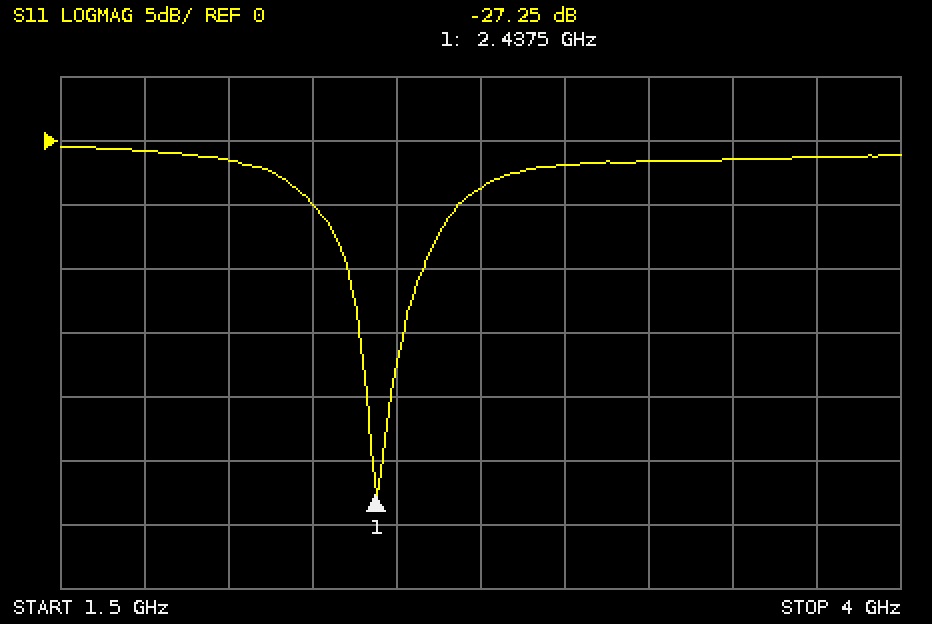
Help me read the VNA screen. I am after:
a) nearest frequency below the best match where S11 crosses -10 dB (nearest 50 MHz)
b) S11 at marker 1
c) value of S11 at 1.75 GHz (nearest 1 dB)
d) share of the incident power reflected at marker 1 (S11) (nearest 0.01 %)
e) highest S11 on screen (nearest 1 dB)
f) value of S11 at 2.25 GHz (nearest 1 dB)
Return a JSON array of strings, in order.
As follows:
["2.35 GHz", "-27.25 dB", "-1 dB", "0.19 %", "0 dB", "-5 dB"]
